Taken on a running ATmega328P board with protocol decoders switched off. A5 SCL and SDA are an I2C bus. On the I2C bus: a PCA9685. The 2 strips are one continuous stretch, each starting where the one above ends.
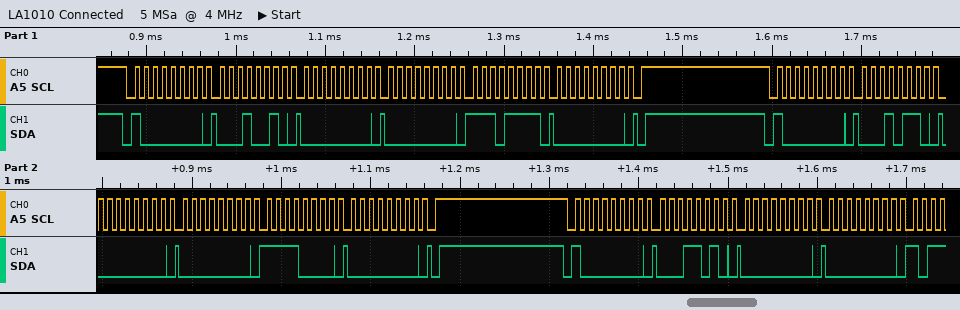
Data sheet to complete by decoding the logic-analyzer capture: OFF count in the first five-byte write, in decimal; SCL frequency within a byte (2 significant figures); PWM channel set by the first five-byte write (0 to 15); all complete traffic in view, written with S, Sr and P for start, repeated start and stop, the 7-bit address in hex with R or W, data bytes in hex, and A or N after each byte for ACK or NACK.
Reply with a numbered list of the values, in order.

1. 239
2. 100 kHz
3. 3
4. S 40W A 12 A 00 A 00 A EF A 00 A P S 40W A 16 A 00 A 00 A F0 A 00 A P S 40W A 1A A 00 A 00 A
